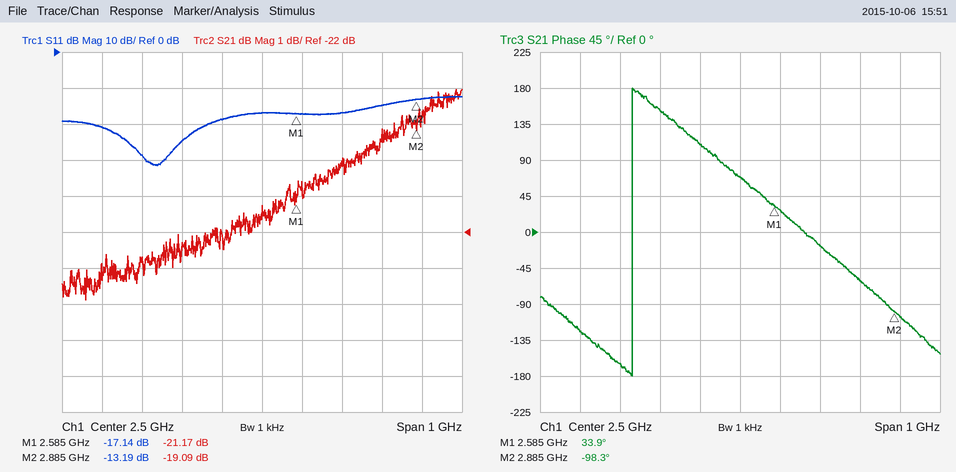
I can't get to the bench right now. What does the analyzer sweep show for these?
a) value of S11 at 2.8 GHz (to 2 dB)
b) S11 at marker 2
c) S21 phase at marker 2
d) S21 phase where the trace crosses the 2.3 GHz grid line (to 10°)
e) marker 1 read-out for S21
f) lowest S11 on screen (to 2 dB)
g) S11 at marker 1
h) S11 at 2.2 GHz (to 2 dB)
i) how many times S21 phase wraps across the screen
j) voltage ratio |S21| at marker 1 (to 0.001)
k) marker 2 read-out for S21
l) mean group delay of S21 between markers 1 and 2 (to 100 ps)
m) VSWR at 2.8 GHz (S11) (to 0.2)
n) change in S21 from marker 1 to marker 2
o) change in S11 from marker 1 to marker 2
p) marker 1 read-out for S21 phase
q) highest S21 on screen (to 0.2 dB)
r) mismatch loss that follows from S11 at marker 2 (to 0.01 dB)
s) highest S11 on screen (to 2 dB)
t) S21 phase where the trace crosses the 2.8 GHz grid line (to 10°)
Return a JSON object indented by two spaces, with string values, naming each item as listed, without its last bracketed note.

{
  "value of S11 at 2.8 GHz": "-14 dB",
  "S11 at marker 2": "-13.19 dB",
  "S21 phase at marker 2": "-98.3°",
  "S21 phase where the trace crosses the 2.3 GHz grid line": "150°",
  "marker 1 read-out for S21": "-21.17 dB",
  "lowest S11 on screen": "-32 dB",
  "S11 at marker 1": "-17.14 dB",
  "S11 at 2.2 GHz": "-28 dB",
  "how many times S21 phase wraps across the screen": "1",
  "voltage ratio |S21| at marker 1": "0.087",
  "marker 2 read-out for S21": "-19.09 dB",
  "mean group delay of S21 between markers 1 and 2": "1.2 ns",
  "VSWR at 2.8 GHz (S11)": "1.4",
  "change in S21 from marker 1 to marker 2": "2.08 dB",
  "change in S11 from marker 1 to marker 2": "3.95 dB",
  "marker 1 read-out for S21 phase": "33.9°",
  "highest S21 on screen": "-18.0 dB",
  "mismatch loss that follows from S11 at marker 2": "0.21 dB",
  "highest S11 on screen": "-12 dB",
  "S21 phase where the trace crosses the 2.8 GHz grid line": "-60°"
}
